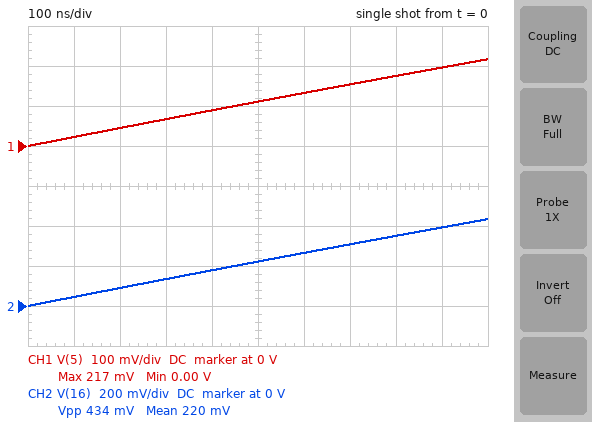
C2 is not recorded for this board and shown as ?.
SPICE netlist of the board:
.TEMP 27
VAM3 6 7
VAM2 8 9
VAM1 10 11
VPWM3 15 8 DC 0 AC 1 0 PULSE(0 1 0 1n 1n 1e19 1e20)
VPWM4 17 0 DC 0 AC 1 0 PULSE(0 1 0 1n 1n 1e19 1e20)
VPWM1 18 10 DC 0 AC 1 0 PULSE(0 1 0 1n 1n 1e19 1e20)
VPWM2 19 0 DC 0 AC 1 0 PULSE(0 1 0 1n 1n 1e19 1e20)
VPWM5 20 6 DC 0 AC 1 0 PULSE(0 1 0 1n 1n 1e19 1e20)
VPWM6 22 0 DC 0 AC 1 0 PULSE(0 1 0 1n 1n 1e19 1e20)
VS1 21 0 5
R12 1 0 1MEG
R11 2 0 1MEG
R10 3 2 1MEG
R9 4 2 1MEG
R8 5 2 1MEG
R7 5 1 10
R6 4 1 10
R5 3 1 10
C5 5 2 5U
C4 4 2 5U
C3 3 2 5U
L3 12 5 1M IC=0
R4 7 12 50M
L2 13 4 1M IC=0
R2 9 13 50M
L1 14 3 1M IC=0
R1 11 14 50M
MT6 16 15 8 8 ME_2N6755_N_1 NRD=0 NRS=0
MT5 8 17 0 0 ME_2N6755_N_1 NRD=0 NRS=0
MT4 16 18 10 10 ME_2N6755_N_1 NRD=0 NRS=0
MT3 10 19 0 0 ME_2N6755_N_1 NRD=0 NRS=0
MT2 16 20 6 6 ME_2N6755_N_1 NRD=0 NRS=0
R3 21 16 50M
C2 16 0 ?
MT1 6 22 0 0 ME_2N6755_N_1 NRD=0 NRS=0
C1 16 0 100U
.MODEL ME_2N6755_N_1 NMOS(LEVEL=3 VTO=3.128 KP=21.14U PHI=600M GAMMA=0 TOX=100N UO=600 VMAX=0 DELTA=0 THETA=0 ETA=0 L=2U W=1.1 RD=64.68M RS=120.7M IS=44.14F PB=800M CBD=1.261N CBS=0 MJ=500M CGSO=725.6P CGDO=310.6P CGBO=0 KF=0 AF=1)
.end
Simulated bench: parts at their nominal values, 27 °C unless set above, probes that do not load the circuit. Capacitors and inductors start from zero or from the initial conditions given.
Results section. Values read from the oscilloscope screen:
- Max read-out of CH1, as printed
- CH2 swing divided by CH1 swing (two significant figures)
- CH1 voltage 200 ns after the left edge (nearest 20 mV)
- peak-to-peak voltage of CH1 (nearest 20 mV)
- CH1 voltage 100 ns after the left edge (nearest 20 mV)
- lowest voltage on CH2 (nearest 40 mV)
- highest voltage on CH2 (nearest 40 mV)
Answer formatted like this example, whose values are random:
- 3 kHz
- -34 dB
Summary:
- 217 mV
- 2.0
- 40 mV
- 220 mV
- 20 mV
- 0 V
- 440 mV
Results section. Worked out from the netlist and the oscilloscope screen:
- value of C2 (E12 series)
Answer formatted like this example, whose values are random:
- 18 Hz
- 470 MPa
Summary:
- 120 µF
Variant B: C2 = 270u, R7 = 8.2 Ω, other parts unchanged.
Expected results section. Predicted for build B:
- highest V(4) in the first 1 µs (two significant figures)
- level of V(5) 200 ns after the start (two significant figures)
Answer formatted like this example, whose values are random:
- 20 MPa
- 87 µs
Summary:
- 130 mV
- 27 mV
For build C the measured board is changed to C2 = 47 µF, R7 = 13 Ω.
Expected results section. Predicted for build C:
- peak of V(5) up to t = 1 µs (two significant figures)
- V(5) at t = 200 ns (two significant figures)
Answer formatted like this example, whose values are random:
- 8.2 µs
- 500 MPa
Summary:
- 320 mV
- 67 mV
